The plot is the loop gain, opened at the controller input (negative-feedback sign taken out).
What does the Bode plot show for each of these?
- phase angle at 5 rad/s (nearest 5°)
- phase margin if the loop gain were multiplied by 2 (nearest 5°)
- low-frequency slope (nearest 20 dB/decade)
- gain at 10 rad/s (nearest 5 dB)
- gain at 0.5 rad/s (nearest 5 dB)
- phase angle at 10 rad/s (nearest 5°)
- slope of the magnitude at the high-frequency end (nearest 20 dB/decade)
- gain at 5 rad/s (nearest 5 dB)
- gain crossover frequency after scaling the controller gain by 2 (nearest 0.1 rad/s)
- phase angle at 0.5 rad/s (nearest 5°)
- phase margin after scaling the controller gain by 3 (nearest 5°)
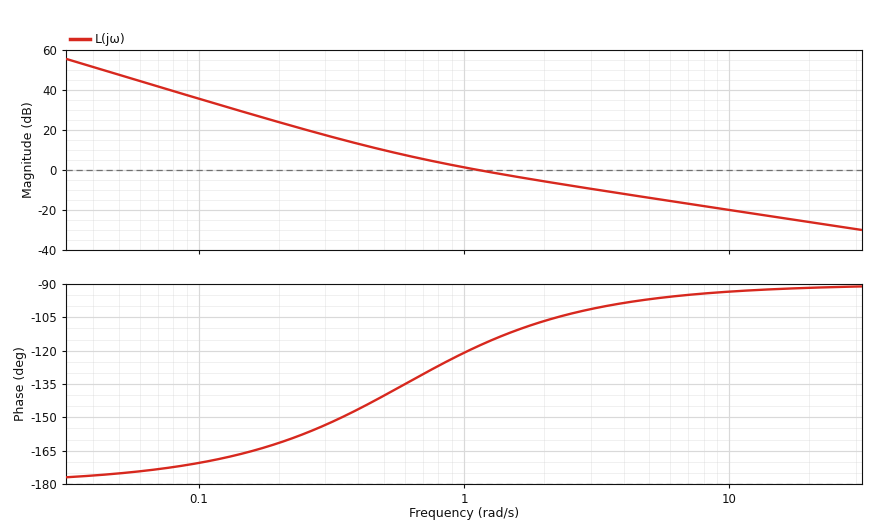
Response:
-95°
75°
-40 dB/decade
-20 dB
10 dB
-95°
-20 dB/decade
-15 dB
2.1 rad/s
-140°
80°
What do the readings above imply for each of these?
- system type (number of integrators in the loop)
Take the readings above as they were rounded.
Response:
2
